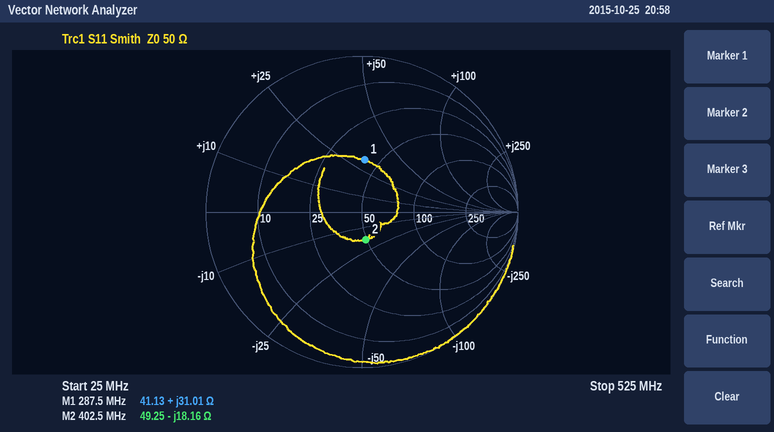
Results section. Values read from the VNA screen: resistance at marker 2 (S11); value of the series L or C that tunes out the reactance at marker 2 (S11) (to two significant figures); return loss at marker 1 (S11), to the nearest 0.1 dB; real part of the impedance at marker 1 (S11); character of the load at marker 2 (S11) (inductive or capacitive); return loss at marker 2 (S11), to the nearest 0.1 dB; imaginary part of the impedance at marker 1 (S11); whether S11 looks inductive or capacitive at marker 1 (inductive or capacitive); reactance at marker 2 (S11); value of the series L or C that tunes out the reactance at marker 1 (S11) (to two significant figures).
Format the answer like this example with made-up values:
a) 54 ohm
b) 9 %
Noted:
a) 49.25 Ω
b) 7.2 nH
c) 9.5 dB
d) 41.13 Ω
e) capacitive
f) 14.9 dB
g) +31.01 Ω
h) inductive
i) -18.16 Ω
j) 18 pF
